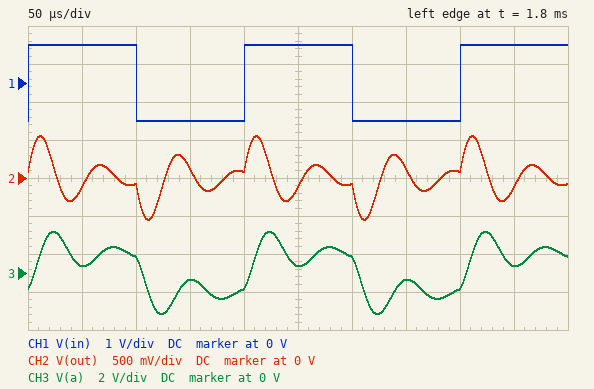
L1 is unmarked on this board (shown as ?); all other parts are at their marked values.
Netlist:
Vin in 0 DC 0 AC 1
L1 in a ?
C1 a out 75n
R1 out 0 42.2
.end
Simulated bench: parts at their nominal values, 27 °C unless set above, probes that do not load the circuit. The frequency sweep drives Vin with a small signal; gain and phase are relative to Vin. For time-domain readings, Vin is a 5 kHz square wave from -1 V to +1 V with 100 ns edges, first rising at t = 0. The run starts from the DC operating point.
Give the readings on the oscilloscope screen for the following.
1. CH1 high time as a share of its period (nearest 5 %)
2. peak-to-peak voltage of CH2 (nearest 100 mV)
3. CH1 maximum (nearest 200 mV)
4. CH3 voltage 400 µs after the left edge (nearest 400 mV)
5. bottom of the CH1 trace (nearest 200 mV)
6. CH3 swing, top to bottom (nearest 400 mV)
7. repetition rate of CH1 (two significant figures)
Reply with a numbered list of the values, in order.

1. 50 %
2. 1.1 V
3. 1.0 V
4. -800 mV
5. -1.0 V
6. 4.4 V
7. 5.0 kHz
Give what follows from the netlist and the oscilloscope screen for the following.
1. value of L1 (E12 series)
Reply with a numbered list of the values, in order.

1. 1 mH
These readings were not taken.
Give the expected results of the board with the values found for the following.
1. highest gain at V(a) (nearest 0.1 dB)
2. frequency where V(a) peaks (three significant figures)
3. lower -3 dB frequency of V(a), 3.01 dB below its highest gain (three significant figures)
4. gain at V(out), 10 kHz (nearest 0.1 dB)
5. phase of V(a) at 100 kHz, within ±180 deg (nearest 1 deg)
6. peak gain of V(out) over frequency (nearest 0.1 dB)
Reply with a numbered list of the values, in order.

1. 9.4 dB
2. 17.8 kHz
3. 14.1 kHz
4. -11.3 dB
5. -113 deg
6. 0 dB
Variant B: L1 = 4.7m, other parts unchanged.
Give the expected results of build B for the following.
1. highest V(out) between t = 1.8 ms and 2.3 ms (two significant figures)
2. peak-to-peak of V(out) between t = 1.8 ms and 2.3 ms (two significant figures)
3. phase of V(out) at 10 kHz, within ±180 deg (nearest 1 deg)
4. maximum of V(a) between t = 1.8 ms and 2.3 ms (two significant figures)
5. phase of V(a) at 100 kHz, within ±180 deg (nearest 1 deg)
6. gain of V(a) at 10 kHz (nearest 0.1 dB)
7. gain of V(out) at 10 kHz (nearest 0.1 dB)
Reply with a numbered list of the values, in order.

1. 210 mV
2. 420 mV
3. -63 deg
4. 2.1 V
5. -116 deg
6. 7.3 dB
7. -6.9 dB
